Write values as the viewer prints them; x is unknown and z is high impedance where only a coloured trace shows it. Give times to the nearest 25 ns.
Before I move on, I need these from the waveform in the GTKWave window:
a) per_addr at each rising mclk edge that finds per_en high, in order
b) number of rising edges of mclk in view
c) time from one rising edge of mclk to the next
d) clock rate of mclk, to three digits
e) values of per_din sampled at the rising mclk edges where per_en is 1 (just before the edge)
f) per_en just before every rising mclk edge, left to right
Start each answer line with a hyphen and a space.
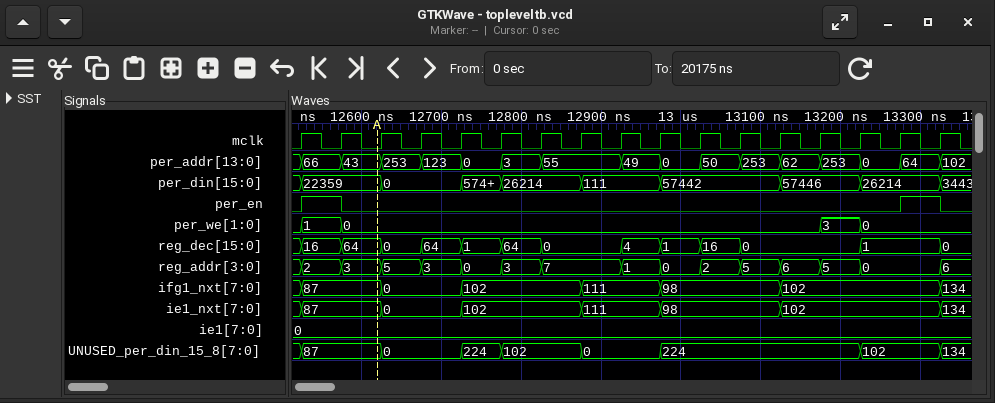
- 66, 64
- 17
- 50 ns
- 20.0 MHz
- 22359, 26214
- 0 1 0 0 0 0 0 0 0 0 0 0 0 0 0 0 1
